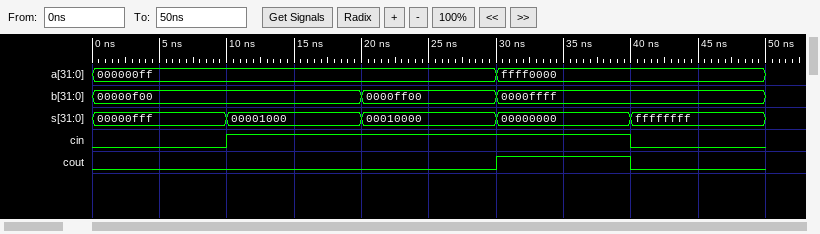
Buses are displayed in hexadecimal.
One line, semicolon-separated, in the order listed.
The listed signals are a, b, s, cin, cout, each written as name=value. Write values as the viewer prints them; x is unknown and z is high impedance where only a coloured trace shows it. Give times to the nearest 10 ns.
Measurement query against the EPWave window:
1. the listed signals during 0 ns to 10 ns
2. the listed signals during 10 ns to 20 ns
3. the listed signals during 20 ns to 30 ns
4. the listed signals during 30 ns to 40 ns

a=000000ff, b=00000f00, s=00000fff, cin=0, cout=0; a=000000ff, b=00000f00, s=00001000, cin=1, cout=0; a=000000ff, b=0000ff00, s=00010000, cin=1, cout=0; a=ffff0000, b=0000ffff, s=00000000, cin=1, cout=1
